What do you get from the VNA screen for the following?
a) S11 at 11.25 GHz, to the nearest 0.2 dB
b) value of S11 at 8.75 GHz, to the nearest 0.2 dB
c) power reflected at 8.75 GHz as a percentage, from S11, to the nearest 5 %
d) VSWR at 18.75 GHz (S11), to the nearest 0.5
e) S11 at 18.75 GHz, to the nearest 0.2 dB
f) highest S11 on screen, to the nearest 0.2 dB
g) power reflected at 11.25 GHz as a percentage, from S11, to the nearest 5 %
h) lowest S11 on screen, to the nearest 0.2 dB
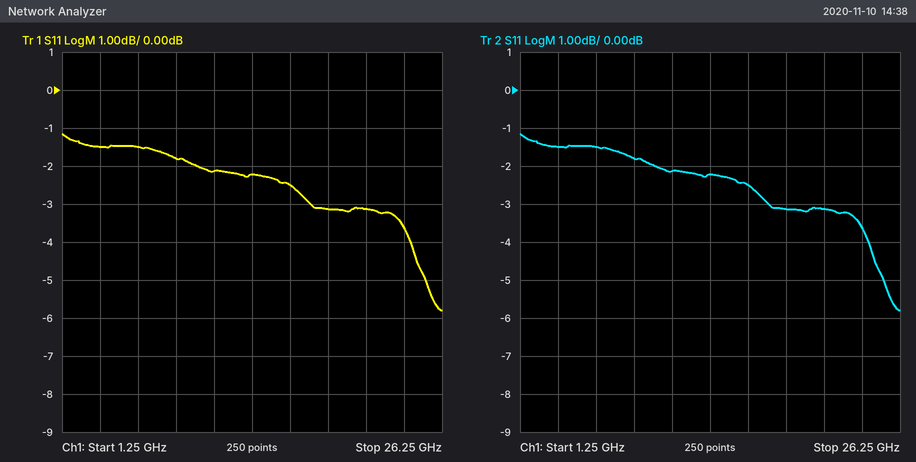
-2.2 dB
-1.8 dB
65 %
5.5
-3.2 dB
-1.2 dB
60 %
-5.8 dB
